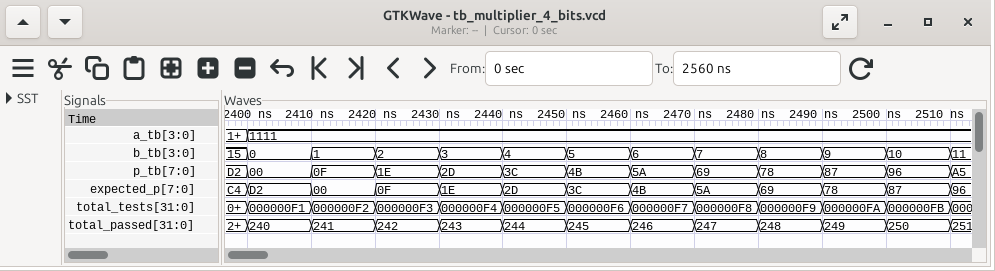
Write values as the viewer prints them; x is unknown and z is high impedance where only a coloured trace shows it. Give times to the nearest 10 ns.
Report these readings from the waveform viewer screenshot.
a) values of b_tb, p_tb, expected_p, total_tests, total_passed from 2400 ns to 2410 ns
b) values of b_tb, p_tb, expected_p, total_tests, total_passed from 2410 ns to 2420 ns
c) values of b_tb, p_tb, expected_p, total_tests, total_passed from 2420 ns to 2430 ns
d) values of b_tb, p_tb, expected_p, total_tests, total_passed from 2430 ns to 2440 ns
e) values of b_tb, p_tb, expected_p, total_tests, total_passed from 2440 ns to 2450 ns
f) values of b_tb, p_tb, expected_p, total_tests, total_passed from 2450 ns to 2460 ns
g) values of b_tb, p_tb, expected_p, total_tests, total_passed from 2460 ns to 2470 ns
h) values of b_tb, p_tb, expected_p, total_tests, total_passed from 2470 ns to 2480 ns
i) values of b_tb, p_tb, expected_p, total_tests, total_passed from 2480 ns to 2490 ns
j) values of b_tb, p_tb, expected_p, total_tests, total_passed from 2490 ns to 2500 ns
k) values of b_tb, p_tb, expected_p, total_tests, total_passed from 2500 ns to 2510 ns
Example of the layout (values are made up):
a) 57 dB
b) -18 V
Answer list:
a) b_tb=0, p_tb=00, expected_p=D2, total_tests=000000F1, total_passed=240
b) b_tb=1, p_tb=0F, expected_p=00, total_tests=000000F2, total_passed=241
c) b_tb=2, p_tb=1E, expected_p=0F, total_tests=000000F3, total_passed=242
d) b_tb=3, p_tb=2D, expected_p=1E, total_tests=000000F4, total_passed=243
e) b_tb=4, p_tb=3C, expected_p=2D, total_tests=000000F5, total_passed=244
f) b_tb=5, p_tb=4B, expected_p=3C, total_tests=000000F6, total_passed=245
g) b_tb=6, p_tb=5A, expected_p=4B, total_tests=000000F7, total_passed=246
h) b_tb=7, p_tb=69, expected_p=5A, total_tests=000000F8, total_passed=247
i) b_tb=8, p_tb=78, expected_p=69, total_tests=000000F9, total_passed=248
j) b_tb=9, p_tb=87, expected_p=78, total_tests=000000FA, total_passed=249
k) b_tb=10, p_tb=96, expected_p=87, total_tests=000000FB, total_passed=250
